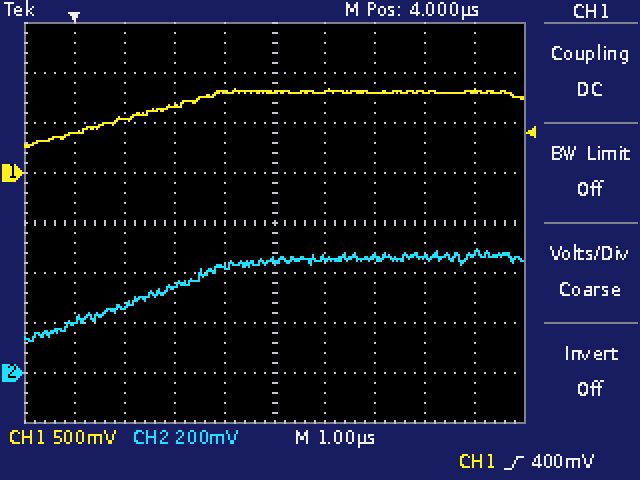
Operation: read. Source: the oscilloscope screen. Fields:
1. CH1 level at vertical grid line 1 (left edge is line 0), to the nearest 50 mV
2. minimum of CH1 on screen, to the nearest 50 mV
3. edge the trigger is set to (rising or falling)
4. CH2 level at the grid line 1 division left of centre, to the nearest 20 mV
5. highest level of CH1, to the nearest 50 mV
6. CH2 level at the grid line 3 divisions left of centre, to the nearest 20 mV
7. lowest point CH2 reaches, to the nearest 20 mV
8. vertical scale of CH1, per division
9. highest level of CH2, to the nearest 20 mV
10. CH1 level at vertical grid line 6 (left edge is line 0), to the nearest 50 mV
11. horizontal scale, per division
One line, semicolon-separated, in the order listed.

400 mV; 250 mV; rising; 420 mV; 850 mV; 260 mV; 120 mV; 500 mV; 500 mV; 800 mV; 1 µs
